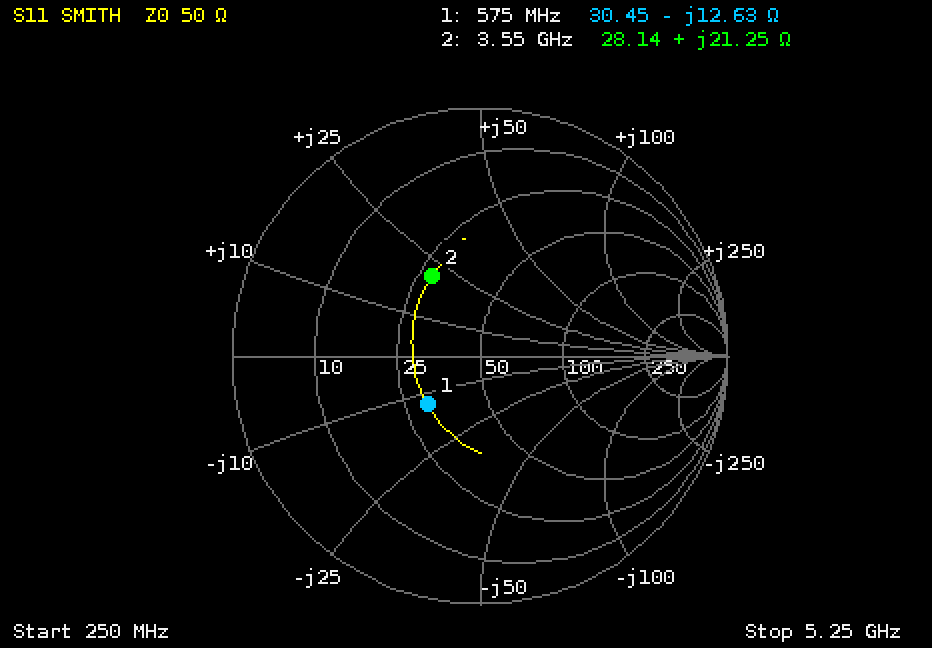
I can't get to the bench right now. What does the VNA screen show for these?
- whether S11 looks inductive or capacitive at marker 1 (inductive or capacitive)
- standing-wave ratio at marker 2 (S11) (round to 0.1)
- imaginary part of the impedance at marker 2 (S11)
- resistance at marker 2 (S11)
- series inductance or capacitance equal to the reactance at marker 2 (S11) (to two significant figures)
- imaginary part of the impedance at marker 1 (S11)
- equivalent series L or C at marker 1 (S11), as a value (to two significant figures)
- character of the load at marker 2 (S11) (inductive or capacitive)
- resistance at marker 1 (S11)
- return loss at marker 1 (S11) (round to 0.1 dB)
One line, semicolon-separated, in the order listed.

capacitive; 2.2; +21.25 Ω; 28.14 Ω; 950 pH; -12.63 Ω; 22 pF; inductive; 30.45 Ω; 10.9 dB
